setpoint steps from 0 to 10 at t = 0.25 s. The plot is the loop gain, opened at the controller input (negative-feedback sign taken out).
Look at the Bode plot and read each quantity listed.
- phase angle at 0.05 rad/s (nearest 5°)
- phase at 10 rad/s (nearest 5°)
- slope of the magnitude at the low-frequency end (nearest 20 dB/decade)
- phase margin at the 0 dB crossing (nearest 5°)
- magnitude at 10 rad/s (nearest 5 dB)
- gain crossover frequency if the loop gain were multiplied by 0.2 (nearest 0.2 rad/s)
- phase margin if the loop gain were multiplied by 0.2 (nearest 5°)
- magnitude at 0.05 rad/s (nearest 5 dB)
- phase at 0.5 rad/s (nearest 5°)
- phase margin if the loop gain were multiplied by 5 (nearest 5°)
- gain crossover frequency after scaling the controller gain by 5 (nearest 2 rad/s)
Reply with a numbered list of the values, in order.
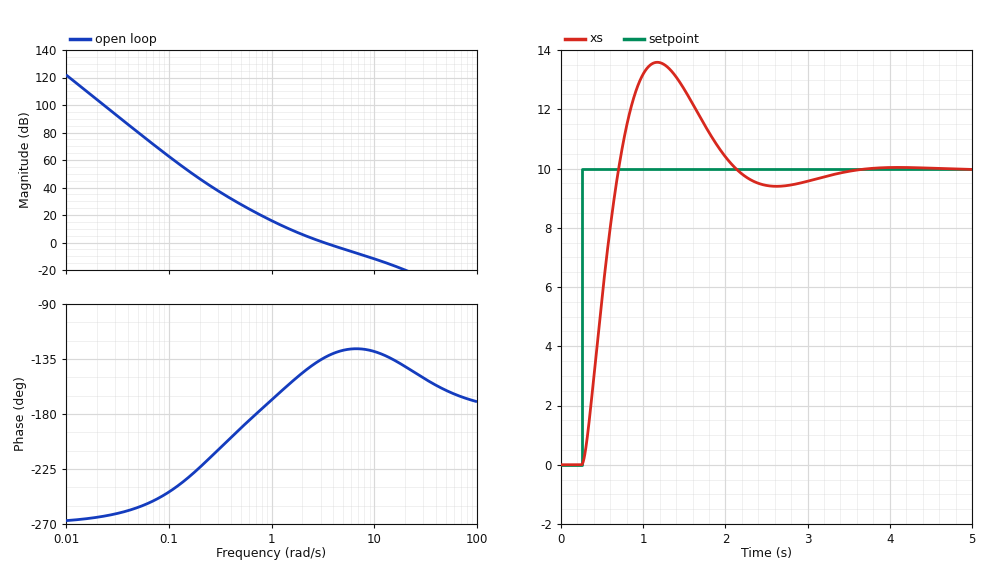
1. -255°
2. -130°
3. -60 dB/decade
4. 45°
5. -10 dB
6. 1.2 rad/s
7. 15°
8. 80 dB
9. -190°
10. 50°
11. 12 rad/s
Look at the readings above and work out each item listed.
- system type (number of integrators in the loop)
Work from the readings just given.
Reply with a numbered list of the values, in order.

1. 3
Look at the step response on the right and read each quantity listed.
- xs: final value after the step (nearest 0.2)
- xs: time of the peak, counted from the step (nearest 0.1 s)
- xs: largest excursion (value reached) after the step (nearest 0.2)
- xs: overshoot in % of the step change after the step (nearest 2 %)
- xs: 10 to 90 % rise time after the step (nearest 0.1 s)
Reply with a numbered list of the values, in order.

1. 10.0
2. 0.9 s
3. 13.6
4. 36 %
5. 0.3 s
